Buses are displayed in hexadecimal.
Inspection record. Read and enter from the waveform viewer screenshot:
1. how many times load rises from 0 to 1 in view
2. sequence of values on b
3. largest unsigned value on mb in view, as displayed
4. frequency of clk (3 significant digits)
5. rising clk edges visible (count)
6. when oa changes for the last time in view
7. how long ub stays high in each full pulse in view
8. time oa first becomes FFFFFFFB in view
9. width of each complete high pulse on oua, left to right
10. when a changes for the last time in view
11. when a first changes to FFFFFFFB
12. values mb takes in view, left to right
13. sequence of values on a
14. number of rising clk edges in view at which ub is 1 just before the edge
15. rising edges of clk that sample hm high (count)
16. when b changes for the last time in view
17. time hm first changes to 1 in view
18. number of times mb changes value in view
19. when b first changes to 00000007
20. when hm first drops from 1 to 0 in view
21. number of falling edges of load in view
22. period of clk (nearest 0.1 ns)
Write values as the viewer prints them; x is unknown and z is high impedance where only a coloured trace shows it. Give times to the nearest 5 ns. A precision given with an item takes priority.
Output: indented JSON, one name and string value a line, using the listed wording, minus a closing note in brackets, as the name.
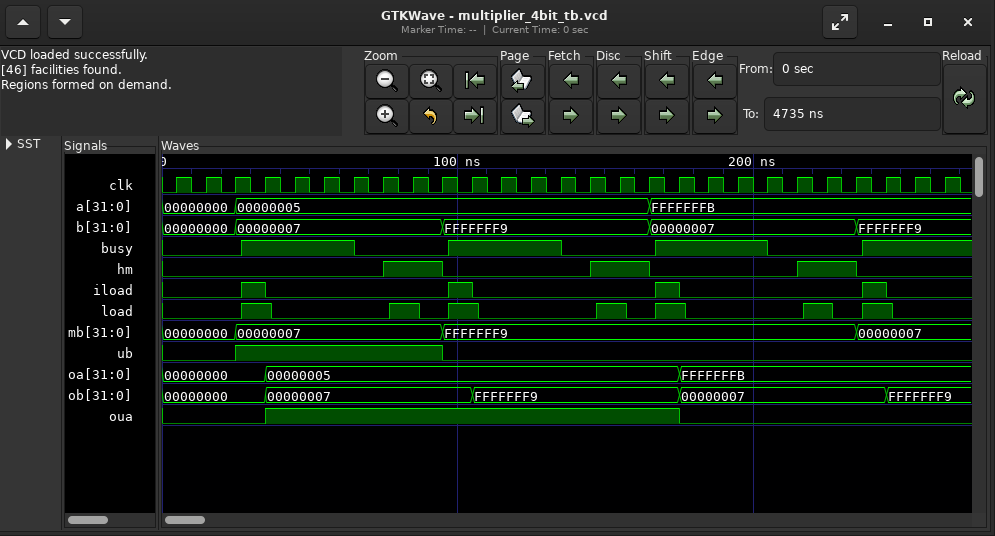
{
  "how many times load rises from 0 to 1 in view": "7",
  "sequence of values on b": "00000000, 00000007, FFFFFFF9, 00000007, FFFFFFF9",
  "largest unsigned value on mb in view, as displayed": "FFFFFFF9",
  "frequency of clk": "100 MHz",
  "rising clk edges visible": "27",
  "when oa changes for the last time in view": "175 ns",
  "how long ub stays high in each full pulse in view": "70 ns",
  "time oa first becomes FFFFFFFB in view": "175 ns",
  "width of each complete high pulse on oua, left to right": "140 ns",
  "when a changes for the last time in view": "165 ns",
  "when a first changes to FFFFFFFB": "165 ns",
  "values mb takes in view, left to right": "00000000, 00000007, FFFFFFF9, 00000007",
  "sequence of values on a": "00000000, 00000005, FFFFFFFB",
  "number of rising clk edges in view at which ub is 1 just before the edge": "7",
  "rising edges of clk that sample hm high": "6",
  "when b changes for the last time in view": "235 ns",
  "time hm first changes to 1 in view": "75 ns",
  "number of times mb changes value in view": "3",
  "when b first changes to 00000007": "25 ns",
  "when hm first drops from 1 to 0 in view": "95 ns",
  "number of falling edges of load in view": "7",
  "period of clk": "10 ns"
}
